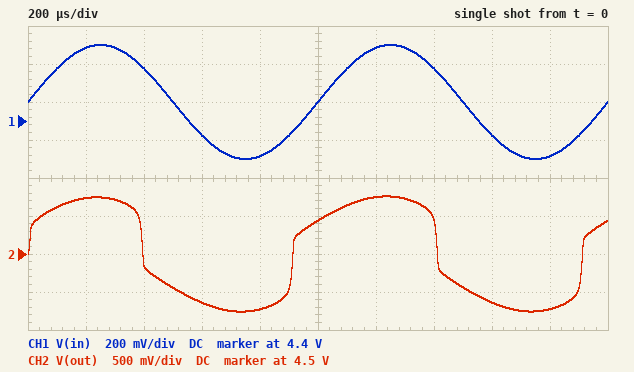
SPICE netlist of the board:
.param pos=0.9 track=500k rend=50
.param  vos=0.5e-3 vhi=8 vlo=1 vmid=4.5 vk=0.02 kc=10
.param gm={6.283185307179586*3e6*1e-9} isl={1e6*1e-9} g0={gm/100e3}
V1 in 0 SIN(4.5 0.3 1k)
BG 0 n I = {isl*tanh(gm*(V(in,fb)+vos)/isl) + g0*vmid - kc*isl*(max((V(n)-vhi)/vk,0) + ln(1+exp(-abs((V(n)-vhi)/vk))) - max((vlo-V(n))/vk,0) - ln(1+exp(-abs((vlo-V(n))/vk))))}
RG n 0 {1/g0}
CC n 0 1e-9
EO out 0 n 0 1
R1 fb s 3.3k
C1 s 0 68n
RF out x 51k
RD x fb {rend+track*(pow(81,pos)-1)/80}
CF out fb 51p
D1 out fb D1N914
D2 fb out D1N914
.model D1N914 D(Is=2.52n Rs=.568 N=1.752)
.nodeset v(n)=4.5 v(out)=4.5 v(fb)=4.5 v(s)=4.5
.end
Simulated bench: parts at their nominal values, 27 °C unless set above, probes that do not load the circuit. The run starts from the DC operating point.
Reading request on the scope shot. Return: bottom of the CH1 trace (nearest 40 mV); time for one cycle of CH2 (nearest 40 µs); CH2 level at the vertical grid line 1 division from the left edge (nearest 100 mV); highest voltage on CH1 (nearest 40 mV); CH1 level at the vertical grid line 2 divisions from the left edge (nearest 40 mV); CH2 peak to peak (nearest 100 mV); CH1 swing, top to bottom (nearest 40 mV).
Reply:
4.20 V
1.00 ms
5.2 V
4.80 V
4.68 V
1.5 V
600 mV
